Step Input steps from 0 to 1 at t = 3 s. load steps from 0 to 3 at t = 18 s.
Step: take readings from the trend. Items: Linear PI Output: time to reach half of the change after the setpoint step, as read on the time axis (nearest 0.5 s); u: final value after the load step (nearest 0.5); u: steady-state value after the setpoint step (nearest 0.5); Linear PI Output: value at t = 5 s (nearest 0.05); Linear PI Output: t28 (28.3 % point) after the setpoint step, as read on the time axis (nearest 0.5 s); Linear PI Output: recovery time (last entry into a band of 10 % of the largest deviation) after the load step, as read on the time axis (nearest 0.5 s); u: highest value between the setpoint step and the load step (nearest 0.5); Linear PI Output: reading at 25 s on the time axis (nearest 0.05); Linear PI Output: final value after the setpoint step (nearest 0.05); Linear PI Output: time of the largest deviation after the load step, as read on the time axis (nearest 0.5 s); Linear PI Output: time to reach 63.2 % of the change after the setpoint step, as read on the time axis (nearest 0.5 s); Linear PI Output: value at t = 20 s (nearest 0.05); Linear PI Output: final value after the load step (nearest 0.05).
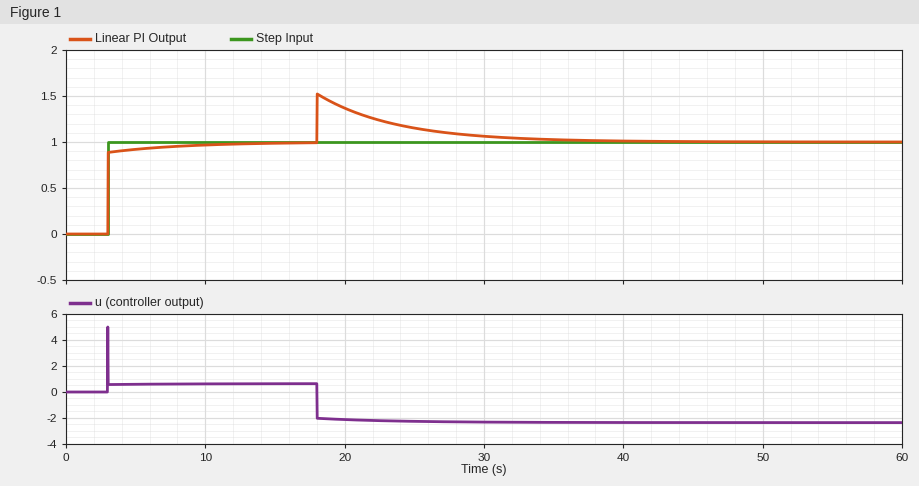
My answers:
3.0 s
-2.5
0.5
0.90
3.0 s
31.0 s
5.0
1.15
1.00
18.0 s
3.0 s
1.35
1.00
